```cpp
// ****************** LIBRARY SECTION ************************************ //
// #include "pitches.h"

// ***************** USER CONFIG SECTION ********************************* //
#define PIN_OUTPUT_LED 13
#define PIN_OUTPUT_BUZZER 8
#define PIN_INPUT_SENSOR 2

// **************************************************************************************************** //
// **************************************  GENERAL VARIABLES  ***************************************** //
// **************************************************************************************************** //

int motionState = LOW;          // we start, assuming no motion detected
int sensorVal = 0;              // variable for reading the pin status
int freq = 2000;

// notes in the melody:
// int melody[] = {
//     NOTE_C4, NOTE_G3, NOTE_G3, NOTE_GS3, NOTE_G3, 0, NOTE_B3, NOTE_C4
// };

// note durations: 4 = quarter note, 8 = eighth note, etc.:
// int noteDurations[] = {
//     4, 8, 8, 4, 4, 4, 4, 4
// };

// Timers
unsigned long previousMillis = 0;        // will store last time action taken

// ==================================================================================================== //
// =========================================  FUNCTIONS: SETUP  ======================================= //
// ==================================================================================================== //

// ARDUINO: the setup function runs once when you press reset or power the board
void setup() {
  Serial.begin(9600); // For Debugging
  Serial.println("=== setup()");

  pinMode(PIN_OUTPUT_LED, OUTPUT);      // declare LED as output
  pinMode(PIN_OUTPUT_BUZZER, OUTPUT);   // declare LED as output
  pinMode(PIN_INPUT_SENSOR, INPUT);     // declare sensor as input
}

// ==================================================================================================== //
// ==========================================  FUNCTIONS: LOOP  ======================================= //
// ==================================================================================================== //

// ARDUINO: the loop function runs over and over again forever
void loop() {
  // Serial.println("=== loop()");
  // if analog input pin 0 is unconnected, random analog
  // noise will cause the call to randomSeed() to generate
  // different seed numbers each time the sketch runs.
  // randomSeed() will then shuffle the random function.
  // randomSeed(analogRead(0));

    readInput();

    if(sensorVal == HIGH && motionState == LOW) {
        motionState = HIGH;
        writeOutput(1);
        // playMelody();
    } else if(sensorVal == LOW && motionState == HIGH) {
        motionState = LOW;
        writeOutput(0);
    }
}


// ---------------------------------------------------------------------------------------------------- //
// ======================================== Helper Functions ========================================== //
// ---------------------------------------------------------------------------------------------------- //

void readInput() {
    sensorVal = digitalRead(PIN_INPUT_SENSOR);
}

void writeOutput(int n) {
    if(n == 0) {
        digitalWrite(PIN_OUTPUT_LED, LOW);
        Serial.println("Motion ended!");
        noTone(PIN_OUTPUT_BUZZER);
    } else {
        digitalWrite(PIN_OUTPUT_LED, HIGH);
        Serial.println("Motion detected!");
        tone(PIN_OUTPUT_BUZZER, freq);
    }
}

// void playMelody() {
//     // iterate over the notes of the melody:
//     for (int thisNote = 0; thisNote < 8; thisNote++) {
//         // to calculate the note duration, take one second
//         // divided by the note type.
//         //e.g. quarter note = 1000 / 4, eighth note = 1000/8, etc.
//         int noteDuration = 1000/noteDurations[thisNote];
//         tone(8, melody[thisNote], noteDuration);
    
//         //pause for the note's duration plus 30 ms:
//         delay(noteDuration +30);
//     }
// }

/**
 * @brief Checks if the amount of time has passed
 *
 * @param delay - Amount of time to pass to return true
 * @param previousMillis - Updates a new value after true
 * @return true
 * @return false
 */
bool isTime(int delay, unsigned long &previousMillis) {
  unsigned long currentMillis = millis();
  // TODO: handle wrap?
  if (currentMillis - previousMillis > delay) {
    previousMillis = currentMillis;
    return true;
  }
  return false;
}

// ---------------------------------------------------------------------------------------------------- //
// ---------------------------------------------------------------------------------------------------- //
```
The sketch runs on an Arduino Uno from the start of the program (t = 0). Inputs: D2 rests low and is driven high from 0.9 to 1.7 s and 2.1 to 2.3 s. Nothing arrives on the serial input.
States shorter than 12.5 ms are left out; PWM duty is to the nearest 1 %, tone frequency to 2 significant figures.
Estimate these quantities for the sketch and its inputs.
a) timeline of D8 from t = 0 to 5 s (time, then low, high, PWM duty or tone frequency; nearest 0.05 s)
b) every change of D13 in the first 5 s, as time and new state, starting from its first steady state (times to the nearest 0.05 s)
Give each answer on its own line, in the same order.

0 s low; 0.9 s tone 2000 Hz; 1.7 s low; 2.1 s tone 2000 Hz; 2.3 s low
0 s low; 0.9 s high; 1.7 s low; 2.1 s high; 2.3 s low
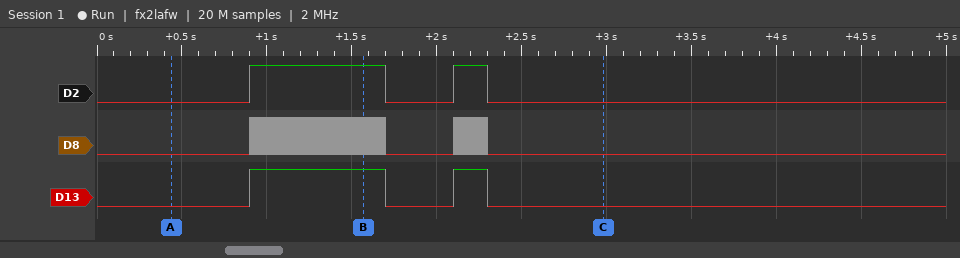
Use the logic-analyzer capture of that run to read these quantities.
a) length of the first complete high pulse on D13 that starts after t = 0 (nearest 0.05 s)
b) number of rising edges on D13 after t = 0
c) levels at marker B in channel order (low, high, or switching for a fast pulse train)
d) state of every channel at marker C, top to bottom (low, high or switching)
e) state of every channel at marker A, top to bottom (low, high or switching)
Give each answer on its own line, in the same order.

0.80 s
2
D2 high, D8 switching, D13 high
D2 low, D8 low, D13 low
D2 low, D8 low, D13 low
